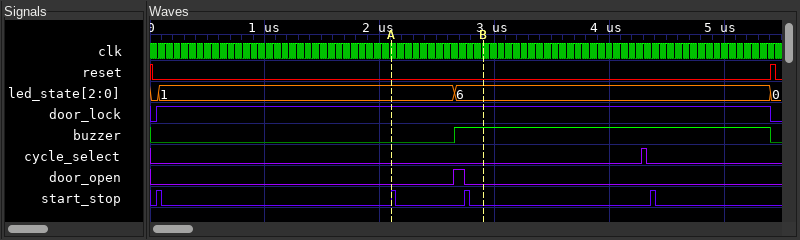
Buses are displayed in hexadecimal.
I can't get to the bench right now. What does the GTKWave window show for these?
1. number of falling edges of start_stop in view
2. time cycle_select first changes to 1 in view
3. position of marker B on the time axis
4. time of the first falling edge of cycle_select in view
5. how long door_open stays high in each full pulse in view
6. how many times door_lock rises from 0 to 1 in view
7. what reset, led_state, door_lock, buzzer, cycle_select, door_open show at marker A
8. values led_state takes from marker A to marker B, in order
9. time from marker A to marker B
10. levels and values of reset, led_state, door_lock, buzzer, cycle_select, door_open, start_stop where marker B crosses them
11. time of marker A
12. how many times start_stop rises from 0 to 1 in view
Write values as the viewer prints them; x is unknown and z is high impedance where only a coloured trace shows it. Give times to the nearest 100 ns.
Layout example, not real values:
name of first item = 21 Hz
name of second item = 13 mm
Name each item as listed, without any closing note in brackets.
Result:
number of falling edges of start_stop in view = 4
time cycle_select first changes to 1 in view = 4300 ns
position of marker B on the time axis = 2900 ns
time of the first falling edge of cycle_select in view = 4300 ns
how long door_open stays high in each full pulse in view = 100 ns
how many times door_lock rises from 0 to 1 in view = 1
what reset, led_state, door_lock, buzzer, cycle_select, door_open show at marker A = reset=0, led_state=1, door_lock=1, buzzer=0, cycle_select=0, door_open=0
values led_state takes from marker A to marker B, in order = 1, 6
time from marker A to marker B = 800 ns
levels and values of reset, led_state, door_lock, buzzer, cycle_select, door_open, start_stop where marker B crosses them = reset=0, led_state=6, door_lock=1, buzzer=1, cycle_select=0, door_open=0, start_stop=0
time of marker A = 2100 ns
how many times start_stop rises from 0 to 1 in view = 4
